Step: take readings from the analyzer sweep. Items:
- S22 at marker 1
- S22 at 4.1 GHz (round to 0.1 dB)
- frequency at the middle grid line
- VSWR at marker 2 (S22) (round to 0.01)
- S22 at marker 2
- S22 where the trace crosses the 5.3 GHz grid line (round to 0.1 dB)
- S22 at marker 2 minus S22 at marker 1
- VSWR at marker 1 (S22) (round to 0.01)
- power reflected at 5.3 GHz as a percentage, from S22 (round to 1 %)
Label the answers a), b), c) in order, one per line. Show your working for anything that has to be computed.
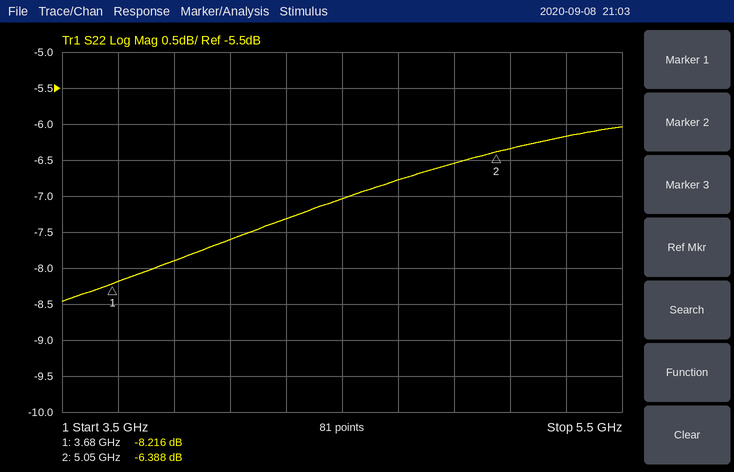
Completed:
a) -8.216 dB
b) -7.6 dB
c) 4.5 GHz
d) (1 + 0.4793)/(1 − 0.4793) ≈ 2.84
e) -6.388 dB
f) -6.2 dB
g) -6.388 − (-8.216) = 1.828 dB
h) (1 + 0.3883)/(1 − 0.3883) ≈ 2.27
i) 10^(-6.2/10) ≈ 24 %
